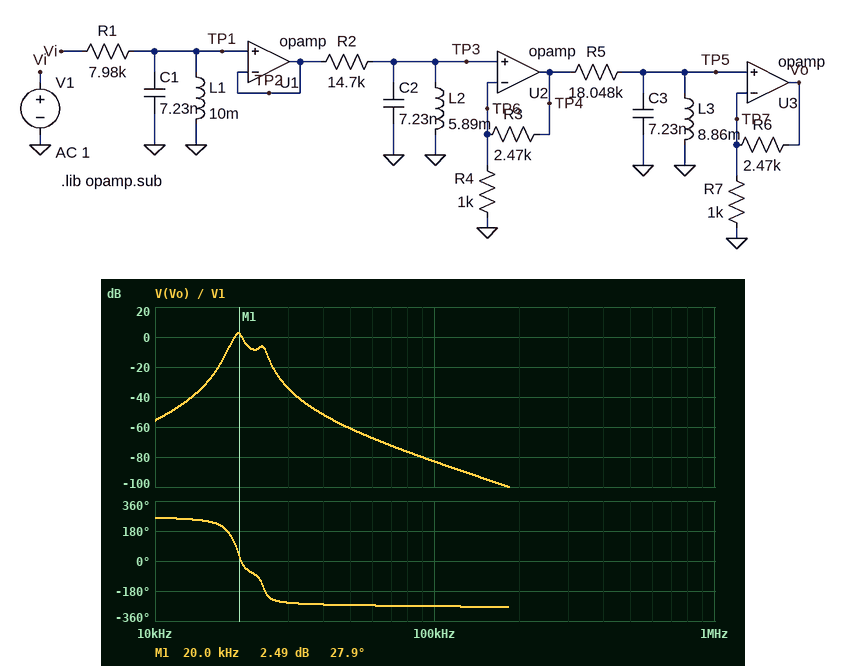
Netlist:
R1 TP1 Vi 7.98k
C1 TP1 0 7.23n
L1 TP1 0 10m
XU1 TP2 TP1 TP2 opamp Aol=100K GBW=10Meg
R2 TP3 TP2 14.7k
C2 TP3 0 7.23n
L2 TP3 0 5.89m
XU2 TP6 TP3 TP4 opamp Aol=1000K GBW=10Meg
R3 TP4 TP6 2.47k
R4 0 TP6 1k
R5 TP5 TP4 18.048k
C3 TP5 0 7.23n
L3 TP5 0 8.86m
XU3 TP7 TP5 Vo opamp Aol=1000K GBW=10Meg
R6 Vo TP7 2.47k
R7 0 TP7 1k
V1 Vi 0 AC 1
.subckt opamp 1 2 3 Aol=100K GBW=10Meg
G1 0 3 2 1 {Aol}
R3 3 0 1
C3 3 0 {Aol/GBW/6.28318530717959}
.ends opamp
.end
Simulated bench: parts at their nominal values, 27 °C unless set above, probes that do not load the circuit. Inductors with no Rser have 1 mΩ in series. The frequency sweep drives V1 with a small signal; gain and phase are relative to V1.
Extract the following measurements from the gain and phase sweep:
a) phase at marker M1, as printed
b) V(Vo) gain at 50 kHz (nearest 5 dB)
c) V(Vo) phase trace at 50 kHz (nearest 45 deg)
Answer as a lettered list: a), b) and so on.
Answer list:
a) 27.9 deg
b) -60 dB
c) -270 deg
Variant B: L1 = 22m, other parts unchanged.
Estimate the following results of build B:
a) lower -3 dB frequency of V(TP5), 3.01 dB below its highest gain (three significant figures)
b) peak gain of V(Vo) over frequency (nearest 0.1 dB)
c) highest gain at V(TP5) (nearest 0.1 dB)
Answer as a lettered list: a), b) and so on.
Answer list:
a) 19.4 kHz
b) -7.9 dB
c) -18.7 dB
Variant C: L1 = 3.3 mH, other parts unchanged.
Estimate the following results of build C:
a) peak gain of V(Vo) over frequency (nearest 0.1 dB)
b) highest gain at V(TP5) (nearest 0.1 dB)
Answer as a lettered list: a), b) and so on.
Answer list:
a) -11.9 dB
b) -22.7 dB
